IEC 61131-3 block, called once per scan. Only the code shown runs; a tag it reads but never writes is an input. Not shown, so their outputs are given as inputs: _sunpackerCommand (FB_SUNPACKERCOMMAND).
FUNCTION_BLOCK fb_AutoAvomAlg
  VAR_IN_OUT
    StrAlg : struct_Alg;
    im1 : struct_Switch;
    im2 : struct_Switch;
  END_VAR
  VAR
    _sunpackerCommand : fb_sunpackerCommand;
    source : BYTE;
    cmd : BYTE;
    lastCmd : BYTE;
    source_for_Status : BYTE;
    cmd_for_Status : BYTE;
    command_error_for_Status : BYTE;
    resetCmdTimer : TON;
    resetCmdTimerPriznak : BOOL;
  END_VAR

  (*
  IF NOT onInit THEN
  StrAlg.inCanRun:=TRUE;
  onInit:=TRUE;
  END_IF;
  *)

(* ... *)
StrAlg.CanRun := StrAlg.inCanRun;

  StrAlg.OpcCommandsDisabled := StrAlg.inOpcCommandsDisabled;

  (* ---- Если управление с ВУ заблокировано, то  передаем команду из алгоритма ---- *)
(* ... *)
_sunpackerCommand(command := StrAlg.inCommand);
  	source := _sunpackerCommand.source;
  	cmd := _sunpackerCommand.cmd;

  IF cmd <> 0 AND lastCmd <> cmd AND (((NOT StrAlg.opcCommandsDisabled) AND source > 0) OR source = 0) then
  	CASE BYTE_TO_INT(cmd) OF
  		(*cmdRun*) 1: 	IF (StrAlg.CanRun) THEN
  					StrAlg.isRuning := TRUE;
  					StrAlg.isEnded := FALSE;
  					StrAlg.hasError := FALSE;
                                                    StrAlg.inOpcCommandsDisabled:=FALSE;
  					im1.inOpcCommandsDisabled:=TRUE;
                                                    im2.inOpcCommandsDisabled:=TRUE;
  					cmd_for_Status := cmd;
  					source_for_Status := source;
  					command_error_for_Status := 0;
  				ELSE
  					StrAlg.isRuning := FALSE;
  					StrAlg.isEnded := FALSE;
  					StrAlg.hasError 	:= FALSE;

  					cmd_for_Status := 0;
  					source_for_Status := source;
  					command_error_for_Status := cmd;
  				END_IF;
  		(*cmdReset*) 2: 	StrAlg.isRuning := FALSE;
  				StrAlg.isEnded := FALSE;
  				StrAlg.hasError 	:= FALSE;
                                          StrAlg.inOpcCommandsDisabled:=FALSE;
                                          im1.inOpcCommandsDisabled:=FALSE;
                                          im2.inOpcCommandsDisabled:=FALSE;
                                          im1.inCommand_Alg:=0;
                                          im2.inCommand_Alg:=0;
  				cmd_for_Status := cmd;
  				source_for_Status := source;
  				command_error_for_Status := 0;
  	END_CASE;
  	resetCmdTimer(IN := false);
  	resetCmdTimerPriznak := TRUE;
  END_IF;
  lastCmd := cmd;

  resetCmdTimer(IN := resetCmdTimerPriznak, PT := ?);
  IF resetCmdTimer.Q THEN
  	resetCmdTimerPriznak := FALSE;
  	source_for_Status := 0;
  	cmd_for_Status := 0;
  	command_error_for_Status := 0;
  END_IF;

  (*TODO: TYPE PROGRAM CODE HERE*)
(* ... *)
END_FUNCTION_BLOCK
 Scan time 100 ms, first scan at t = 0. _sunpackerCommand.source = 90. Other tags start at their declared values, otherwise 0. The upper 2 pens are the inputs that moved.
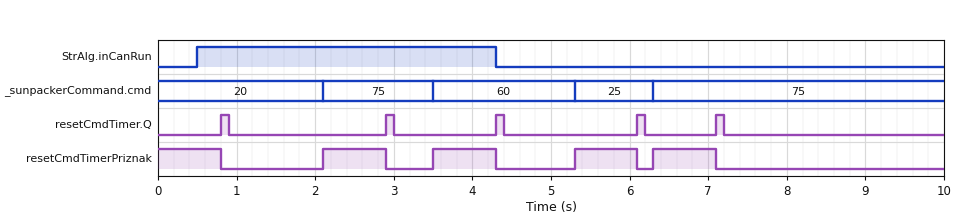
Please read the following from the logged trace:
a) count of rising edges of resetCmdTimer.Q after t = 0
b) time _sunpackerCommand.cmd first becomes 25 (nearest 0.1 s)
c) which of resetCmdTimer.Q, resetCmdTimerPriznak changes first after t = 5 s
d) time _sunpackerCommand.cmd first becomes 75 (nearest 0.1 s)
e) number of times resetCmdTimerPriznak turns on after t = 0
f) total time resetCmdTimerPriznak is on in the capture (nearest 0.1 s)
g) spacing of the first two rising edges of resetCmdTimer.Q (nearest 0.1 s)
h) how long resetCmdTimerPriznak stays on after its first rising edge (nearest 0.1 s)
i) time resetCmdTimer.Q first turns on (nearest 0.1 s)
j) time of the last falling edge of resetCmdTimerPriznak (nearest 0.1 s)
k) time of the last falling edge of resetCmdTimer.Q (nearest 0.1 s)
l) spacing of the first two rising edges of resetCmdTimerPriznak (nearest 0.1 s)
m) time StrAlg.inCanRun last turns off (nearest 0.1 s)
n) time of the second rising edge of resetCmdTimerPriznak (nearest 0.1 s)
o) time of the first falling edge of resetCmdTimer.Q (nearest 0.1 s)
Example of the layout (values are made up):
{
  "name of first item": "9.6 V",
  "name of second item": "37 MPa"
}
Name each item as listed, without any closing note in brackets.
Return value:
{
  "count of rising edges of resetCmdTimer.Q after t = 0": "5",
  "time _sunpackerCommand.cmd first becomes 25": "5.3 s",
  "which of resetCmdTimer.Q, resetCmdTimerPriznak changes first after t = 5 s": "resetCmdTimerPriznak",
  "time _sunpackerCommand.cmd first becomes 75": "2.1 s",
  "number of times resetCmdTimerPriznak turns on after t = 0": "4",
  "total time resetCmdTimerPriznak is on in the capture": "4.0 s",
  "spacing of the first two rising edges of resetCmdTimer.Q": "2.1 s",
  "how long resetCmdTimerPriznak stays on after its first rising edge": "0.8 s",
  "time resetCmdTimer.Q first turns on": "0.8 s",
  "time of the last falling edge of resetCmdTimerPriznak": "7.1 s",
  "time of the last falling edge of resetCmdTimer.Q": "7.2 s",
  "spacing of the first two rising edges of resetCmdTimerPriznak": "1.4 s",
  "time StrAlg.inCanRun last turns off": "4.3 s",
  "time of the second rising edge of resetCmdTimerPriznak": "3.5 s",
  "time of the first falling edge of resetCmdTimer.Q": "0.9 s"
}
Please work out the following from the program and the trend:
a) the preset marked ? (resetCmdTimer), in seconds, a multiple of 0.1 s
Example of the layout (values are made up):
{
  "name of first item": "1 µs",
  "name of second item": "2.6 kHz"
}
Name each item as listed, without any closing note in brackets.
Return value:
{
  "the preset marked ? (resetCmdTimer), in seconds, a multiple of 0.1 s": "0.8 s"
}
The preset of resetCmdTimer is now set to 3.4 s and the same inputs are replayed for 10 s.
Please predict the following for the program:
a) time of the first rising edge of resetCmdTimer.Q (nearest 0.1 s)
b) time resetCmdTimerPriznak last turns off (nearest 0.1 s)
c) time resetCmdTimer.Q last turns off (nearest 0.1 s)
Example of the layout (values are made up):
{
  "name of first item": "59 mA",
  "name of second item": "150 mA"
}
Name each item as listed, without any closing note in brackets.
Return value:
{
  "time of the first rising edge of resetCmdTimer.Q": "9.7 s",
  "time resetCmdTimerPriznak last turns off": "9.7 s",
  "time resetCmdTimer.Q last turns off": "9.8 s"
}
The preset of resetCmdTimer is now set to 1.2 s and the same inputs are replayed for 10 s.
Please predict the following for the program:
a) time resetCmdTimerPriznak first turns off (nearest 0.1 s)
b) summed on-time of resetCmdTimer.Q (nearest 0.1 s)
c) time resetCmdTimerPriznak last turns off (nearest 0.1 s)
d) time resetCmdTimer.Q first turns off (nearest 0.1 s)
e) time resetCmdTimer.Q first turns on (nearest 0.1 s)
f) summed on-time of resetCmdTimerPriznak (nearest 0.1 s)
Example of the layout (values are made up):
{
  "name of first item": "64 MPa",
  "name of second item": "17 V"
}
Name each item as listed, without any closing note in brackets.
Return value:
{
  "time resetCmdTimerPriznak first turns off": "1.2 s",
  "summed on-time of resetCmdTimer.Q": "0.4 s",
  "time resetCmdTimerPriznak last turns off": "7.5 s",
  "time resetCmdTimer.Q first turns off": "1.3 s",
  "time resetCmdTimer.Q first turns on": "1.2 s",
  "summed on-time of resetCmdTimerPriznak": "5.8 s"
}
